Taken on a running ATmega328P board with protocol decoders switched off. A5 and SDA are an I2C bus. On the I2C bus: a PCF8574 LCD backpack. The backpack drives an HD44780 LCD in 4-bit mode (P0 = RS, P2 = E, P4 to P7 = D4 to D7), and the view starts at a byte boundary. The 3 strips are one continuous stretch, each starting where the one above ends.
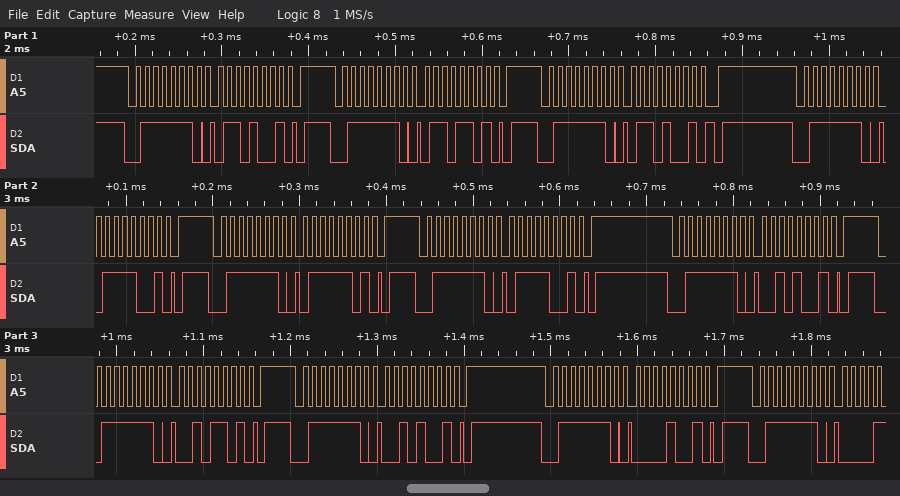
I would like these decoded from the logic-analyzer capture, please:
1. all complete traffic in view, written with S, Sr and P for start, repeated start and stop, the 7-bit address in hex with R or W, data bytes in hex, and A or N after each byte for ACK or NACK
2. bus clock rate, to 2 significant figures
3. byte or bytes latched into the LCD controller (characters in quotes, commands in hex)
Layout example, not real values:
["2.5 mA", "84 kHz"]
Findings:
["S 3FW A 69 A P S 3FW A 6D A P S 3FW A 69 A P S 3FW A 79 A P S 3FW A 7D A P S 3FW A 79 A P S 3FW A 29 A P S 3FW A 2D A P S 3FW A 29 A P S 3FW A 09 A P S 3FW A", "100 kHz", "'g'"]
